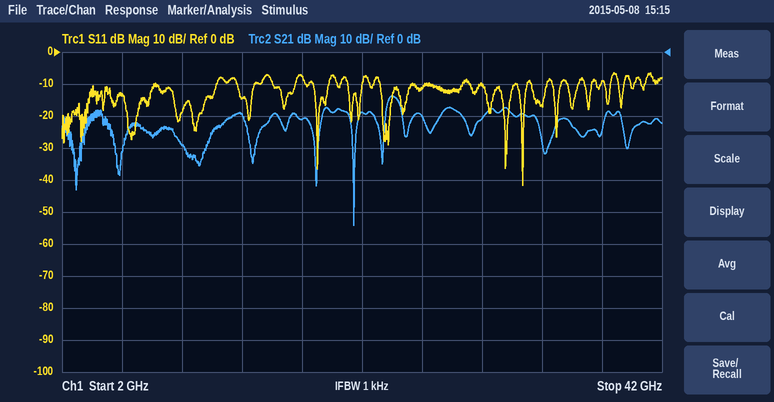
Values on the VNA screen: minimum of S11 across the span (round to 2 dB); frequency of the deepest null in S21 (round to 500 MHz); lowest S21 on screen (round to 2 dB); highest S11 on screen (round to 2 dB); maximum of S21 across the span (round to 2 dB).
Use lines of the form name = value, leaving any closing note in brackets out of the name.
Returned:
minimum of S11 across the span = -42 dB
frequency of the deepest null in S21 = 21.5 GHz
lowest S21 on screen = -54 dB
highest S11 on screen = -6 dB
maximum of S21 across the span = -14 dB
